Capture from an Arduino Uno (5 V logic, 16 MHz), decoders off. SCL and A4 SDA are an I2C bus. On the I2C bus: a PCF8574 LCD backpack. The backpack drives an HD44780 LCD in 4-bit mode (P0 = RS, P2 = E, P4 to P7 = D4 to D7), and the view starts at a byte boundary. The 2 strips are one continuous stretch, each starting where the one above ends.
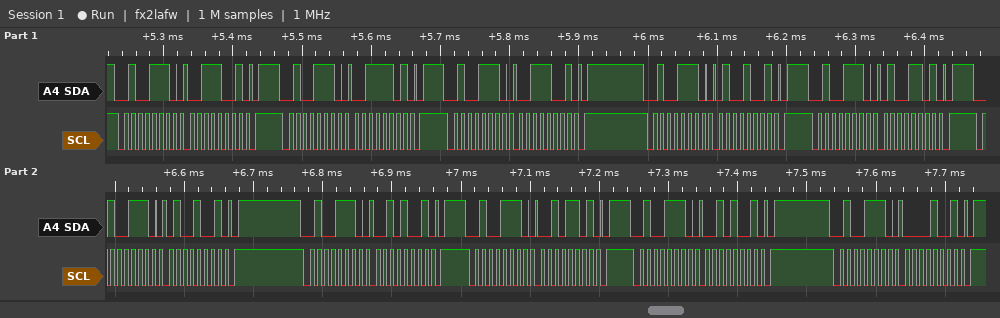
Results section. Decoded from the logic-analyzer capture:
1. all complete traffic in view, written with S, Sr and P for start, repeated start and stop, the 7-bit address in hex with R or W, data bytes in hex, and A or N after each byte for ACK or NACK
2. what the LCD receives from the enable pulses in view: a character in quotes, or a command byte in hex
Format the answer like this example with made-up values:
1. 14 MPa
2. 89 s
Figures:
1. S 27W A 39 A P S 27W A 3D A P S 27W A 39 A P S 27W A 49 A P S 27W A 4D A P S 27W A 49 A P S 27W A 29 A P S 27W A 2D A P S 27W A 29 A P S 27W A 09 A P
2. '4'
